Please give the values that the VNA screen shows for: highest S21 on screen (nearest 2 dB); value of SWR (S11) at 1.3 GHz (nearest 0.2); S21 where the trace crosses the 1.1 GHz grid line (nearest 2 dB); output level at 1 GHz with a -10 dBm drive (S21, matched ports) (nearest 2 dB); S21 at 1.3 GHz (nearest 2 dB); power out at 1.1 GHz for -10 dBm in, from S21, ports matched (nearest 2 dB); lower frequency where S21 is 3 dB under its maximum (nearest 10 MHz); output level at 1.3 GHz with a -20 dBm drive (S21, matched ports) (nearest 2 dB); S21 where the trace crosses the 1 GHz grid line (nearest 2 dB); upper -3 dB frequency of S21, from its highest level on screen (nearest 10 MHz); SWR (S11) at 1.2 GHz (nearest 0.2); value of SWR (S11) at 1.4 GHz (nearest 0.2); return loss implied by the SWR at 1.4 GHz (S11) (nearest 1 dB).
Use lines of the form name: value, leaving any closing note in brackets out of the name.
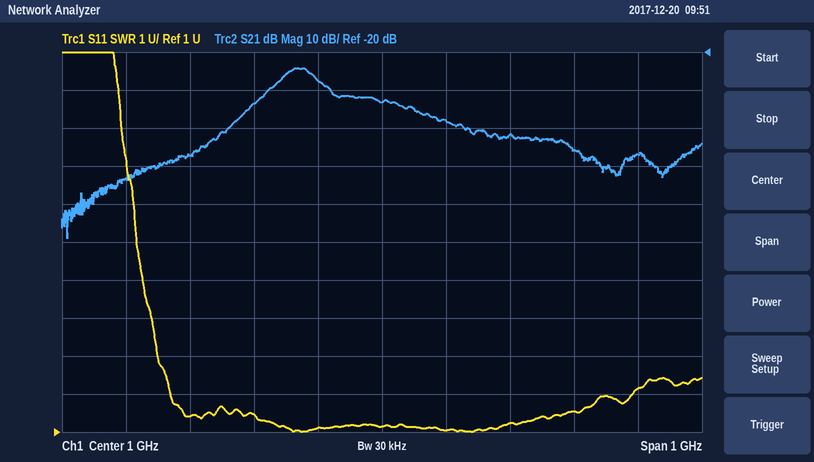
highest S21 on screen: -24 dB
value of SWR (S11) at 1.3 GHz: 1.6
S21 where the trace crosses the 1.1 GHz grid line: -38 dB
output level at 1 GHz with a -10 dBm drive (S21, matched ports): -44 dBm
S21 at 1.3 GHz: -46 dB
power out at 1.1 GHz for -10 dBm in, from S21, ports matched: -48 dBm
lower frequency where S21 is 3 dB under its maximum: 840 MHz
output level at 1.3 GHz with a -20 dBm drive (S21, matched ports): -66 dBm
S21 where the trace crosses the 1 GHz grid line: -34 dB
upper -3 dB frequency of S21, from its highest level on screen: 900 MHz
SWR (S11) at 1.2 GHz: 1.2
value of SWR (S11) at 1.4 GHz: 2.2
return loss implied by the SWR at 1.4 GHz (S11): 9 dB
